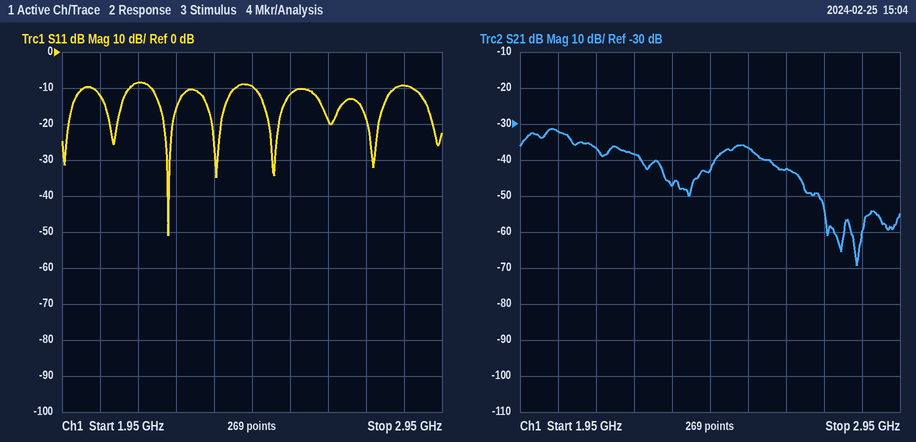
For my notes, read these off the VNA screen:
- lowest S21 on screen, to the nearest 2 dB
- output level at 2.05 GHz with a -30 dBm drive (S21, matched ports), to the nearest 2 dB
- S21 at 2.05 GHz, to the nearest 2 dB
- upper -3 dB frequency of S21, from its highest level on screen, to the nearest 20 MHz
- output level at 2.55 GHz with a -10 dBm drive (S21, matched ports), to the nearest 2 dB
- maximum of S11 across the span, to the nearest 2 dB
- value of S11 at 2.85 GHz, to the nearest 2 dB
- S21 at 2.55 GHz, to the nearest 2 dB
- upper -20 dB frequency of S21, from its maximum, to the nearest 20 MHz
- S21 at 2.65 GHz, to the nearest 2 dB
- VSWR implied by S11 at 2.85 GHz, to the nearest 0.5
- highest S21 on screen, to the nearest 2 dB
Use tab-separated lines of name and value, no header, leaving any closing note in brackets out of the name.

lowest S21 on screen, to the nearest 2 dB	-70 dB
output level at 2.05 GHz with a -30 dBm drive (S21, matched ports), to the nearest 2 dB	-62 dBm
S21 at 2.05 GHz, to the nearest 2 dB	-32 dB
upper -3 dB frequency of S21, from its highest level on screen, to the nearest 20 MHz	2.08 GHz
output level at 2.55 GHz with a -10 dBm drive (S21, matched ports), to the nearest 2 dB	-46 dBm
maximum of S11 across the span, to the nearest 2 dB	-8 dB
value of S11 at 2.85 GHz, to the nearest 2 dB	-10 dB
S21 at 2.55 GHz, to the nearest 2 dB	-36 dB
upper -20 dB frequency of S21, from its maximum, to the nearest 20 MHz	2.74 GHz
S21 at 2.65 GHz, to the nearest 2 dB	-42 dB
VSWR implied by S11 at 2.85 GHz, to the nearest 0.5	2.0
highest S21 on screen, to the nearest 2 dB	-32 dB
